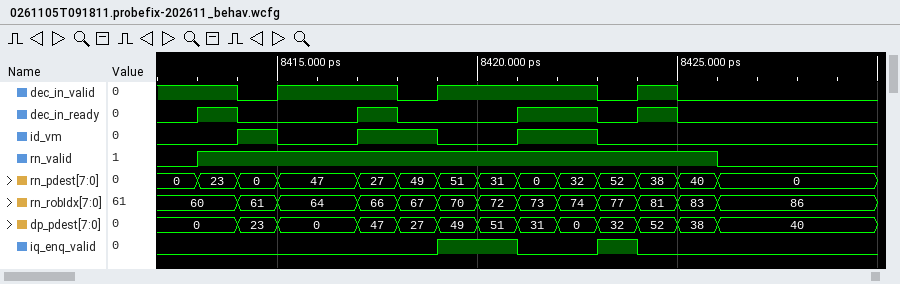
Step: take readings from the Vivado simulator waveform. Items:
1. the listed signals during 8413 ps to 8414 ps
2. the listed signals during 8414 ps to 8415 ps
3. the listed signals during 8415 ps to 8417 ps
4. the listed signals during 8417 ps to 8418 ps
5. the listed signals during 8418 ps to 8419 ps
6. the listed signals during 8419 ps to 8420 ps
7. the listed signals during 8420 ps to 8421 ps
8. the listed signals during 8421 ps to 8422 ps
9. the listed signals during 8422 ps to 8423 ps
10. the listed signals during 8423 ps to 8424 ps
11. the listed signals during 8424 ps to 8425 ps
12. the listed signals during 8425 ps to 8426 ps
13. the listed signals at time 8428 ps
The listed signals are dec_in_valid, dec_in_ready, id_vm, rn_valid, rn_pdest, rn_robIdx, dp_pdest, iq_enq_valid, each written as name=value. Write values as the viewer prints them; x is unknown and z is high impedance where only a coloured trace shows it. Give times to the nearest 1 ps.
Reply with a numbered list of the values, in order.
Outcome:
1. dec_in_valid=1, dec_in_ready=1, id_vm=0, rn_valid=1, rn_pdest=23, rn_robIdx=60, dp_pdest=0, iq_enq_valid=0
2. dec_in_valid=0, dec_in_ready=0, id_vm=1, rn_valid=1, rn_pdest=0, rn_robIdx=61, dp_pdest=23, iq_enq_valid=0
3. dec_in_valid=1, dec_in_ready=0, id_vm=0, rn_valid=1, rn_pdest=47, rn_robIdx=64, dp_pdest=0, iq_enq_valid=0
4. dec_in_valid=1, dec_in_ready=1, id_vm=1, rn_valid=1, rn_pdest=27, rn_robIdx=66, dp_pdest=47, iq_enq_valid=0
5. dec_in_valid=0, dec_in_ready=0, id_vm=1, rn_valid=1, rn_pdest=49, rn_robIdx=67, dp_pdest=27, iq_enq_valid=0
6. dec_in_valid=1, dec_in_ready=0, id_vm=0, rn_valid=1, rn_pdest=51, rn_robIdx=70, dp_pdest=49, iq_enq_valid=1
7. dec_in_valid=1, dec_in_ready=0, id_vm=0, rn_valid=1, rn_pdest=31, rn_robIdx=72, dp_pdest=51, iq_enq_valid=1
8. dec_in_valid=1, dec_in_ready=1, id_vm=1, rn_valid=1, rn_pdest=0, rn_robIdx=73, dp_pdest=31, iq_enq_valid=0
9. dec_in_valid=1, dec_in_ready=1, id_vm=1, rn_valid=1, rn_pdest=32, rn_robIdx=74, dp_pdest=0, iq_enq_valid=0
10. dec_in_valid=0, dec_in_ready=0, id_vm=0, rn_valid=1, rn_pdest=52, rn_robIdx=77, dp_pdest=32, iq_enq_valid=1
11. dec_in_valid=1, dec_in_ready=1, id_vm=0, rn_valid=1, rn_pdest=38, rn_robIdx=81, dp_pdest=52, iq_enq_valid=0
12. dec_in_valid=0, dec_in_ready=0, id_vm=0, rn_valid=1, rn_pdest=40, rn_robIdx=83, dp_pdest=38, iq_enq_valid=0
13. dec_in_valid=0, dec_in_ready=0, id_vm=0, rn_valid=0, rn_pdest=0, rn_robIdx=86, dp_pdest=40, iq_enq_valid=0
